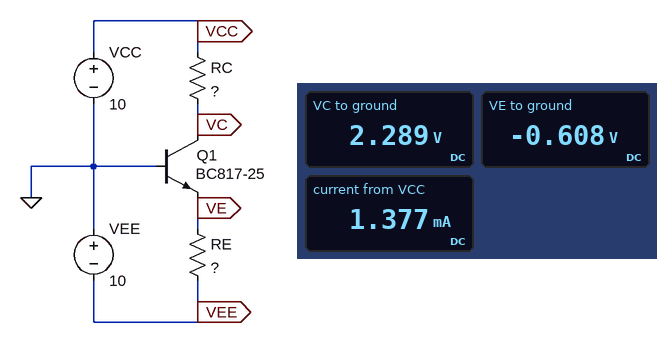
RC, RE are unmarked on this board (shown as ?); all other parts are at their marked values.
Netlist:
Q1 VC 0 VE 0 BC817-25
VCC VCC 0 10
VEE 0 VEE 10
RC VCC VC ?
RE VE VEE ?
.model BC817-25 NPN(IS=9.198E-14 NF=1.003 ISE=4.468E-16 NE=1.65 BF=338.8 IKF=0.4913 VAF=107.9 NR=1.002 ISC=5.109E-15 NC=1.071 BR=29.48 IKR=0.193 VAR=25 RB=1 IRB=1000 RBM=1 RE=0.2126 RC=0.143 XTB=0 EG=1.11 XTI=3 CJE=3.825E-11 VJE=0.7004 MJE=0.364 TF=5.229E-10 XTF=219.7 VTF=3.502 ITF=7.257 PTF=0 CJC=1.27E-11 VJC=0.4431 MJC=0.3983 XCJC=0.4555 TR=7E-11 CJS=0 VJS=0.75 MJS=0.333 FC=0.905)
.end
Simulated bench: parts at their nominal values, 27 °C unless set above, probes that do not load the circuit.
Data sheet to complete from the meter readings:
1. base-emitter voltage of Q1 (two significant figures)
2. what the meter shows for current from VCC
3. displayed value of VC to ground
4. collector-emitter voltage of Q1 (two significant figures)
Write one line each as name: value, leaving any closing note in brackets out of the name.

base-emitter voltage of Q1: 610 mV
what the meter shows for current from VCC: 1.377 mA
displayed value of VC to ground: 2.289 V
collector-emitter voltage of Q1: 2.9 V
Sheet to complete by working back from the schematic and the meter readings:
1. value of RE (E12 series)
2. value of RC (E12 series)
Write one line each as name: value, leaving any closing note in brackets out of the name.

value of RE: 6.8 kΩ
value of RC: 5.6 kΩ
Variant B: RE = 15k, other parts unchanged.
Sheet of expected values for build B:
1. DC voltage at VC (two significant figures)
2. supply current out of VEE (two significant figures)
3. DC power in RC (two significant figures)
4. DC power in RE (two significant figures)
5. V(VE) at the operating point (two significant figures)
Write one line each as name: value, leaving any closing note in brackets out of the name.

DC voltage at VC: 6.5 V
supply current out of VEE: 630 µA
DC power in RC: 2.2 mW
DC power in RE: 5.9 mW
V(VE) at the operating point: -590 mV
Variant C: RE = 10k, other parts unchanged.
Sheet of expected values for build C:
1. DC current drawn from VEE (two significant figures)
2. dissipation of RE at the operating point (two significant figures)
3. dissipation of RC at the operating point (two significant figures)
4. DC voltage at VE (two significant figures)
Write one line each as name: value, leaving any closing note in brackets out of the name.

DC current drawn from VEE: 940 µA
dissipation of RE at the operating point: 8.8 mW
dissipation of RC at the operating point: 4.9 mW
DC voltage at VE: -600 mV
